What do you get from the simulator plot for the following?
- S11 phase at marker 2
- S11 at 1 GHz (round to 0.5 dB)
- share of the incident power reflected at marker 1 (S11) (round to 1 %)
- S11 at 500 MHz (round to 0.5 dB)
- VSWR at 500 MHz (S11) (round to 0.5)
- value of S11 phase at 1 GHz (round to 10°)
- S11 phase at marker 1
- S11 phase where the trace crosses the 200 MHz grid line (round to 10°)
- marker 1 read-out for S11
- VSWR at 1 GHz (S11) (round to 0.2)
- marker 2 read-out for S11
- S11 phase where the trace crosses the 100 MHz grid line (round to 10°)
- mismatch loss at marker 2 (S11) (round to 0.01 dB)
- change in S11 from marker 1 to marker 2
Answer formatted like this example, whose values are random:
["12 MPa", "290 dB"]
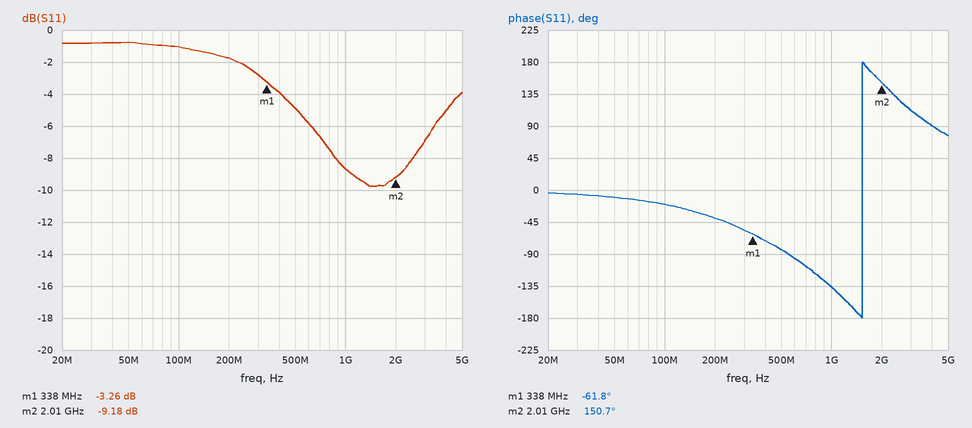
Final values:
["150.7°", "-8.5 dB", "47 %", "-5.0 dB", "3.5", "-140°", "-61.8°", "-40°", "-3.26 dB", "2.2", "-9.18 dB", "-20°", "0.56 dB", "-5.92 dB"]
